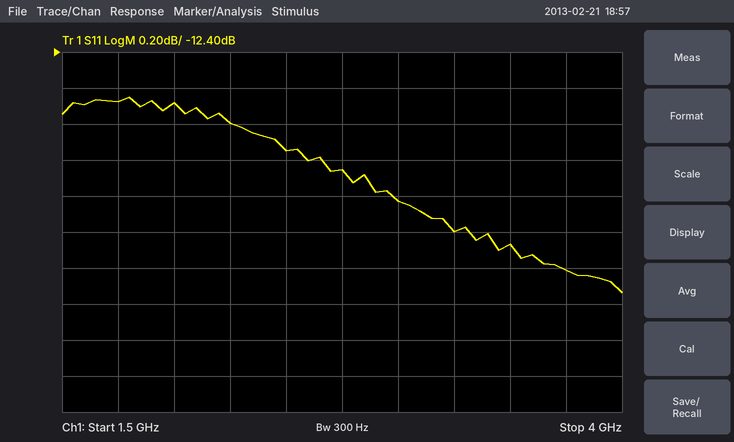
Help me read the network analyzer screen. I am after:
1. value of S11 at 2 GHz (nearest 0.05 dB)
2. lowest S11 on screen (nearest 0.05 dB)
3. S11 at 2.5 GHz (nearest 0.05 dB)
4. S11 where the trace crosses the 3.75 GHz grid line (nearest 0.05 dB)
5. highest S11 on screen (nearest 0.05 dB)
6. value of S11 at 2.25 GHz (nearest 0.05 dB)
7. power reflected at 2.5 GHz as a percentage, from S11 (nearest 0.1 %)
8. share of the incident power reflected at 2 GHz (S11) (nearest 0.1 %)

-12.70 dB
-13.75 dB
-12.95 dB
-13.60 dB
-12.65 dB
-12.80 dB
5.1 %
5.4 %
